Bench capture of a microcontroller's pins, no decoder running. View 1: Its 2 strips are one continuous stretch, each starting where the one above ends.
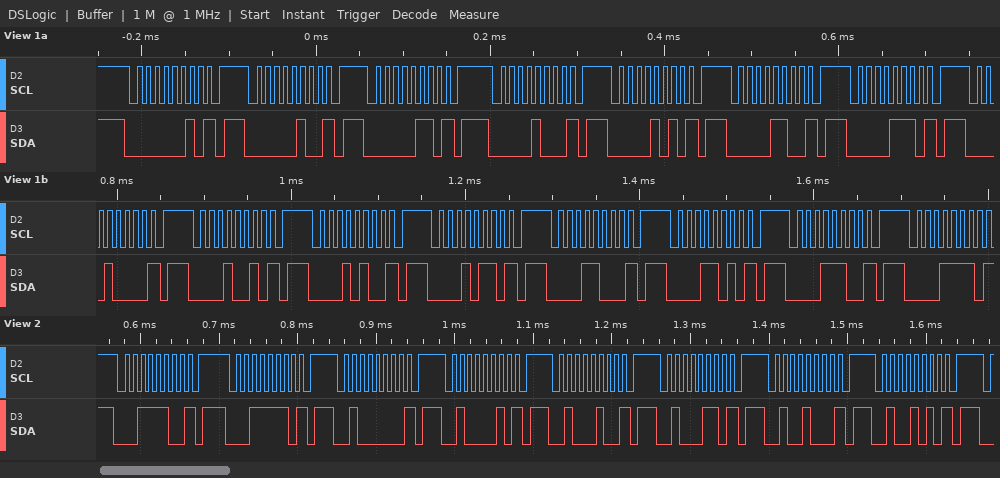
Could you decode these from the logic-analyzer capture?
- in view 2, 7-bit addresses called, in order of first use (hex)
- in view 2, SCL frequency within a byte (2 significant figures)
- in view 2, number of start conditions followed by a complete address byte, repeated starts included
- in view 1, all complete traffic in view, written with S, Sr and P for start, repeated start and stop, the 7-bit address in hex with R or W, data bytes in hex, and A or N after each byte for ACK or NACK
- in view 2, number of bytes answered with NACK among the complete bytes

0x1E 0x1F 0x20 0x21 0x22 0x23 0x24 0x25
100 kHz
8
S 01W N P S 02W N P S 03W N P S 04W N P S 05W N P S 06W N P S 07W N P S 08W N P S 09W N P S 0AW N P S 0BW N P S 0CW N P S 0DW N P S 0EW N P S 0FW N
8
